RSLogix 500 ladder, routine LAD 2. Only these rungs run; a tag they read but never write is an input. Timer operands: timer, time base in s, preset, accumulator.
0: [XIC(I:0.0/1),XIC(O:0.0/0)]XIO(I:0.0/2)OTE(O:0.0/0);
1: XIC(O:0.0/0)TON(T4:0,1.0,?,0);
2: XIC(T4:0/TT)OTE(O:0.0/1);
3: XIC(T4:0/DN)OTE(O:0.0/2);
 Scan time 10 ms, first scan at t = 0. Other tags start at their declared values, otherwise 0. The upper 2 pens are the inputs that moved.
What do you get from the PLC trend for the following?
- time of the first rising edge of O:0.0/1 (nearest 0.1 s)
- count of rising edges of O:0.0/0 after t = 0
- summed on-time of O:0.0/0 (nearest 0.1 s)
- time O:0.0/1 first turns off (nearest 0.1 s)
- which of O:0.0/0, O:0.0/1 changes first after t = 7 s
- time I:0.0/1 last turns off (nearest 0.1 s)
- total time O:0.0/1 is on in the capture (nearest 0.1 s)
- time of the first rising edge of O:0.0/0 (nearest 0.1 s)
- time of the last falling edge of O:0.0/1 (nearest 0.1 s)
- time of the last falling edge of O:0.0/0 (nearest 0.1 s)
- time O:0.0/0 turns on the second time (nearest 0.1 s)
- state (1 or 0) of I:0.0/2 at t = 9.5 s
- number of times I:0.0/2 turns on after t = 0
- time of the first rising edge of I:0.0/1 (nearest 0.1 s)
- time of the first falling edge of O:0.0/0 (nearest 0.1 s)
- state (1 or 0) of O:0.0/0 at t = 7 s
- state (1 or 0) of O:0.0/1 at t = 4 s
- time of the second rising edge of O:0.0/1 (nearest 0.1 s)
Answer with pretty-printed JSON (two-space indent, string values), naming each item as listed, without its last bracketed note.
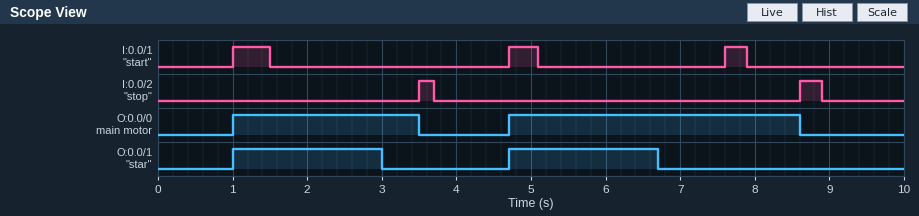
{
  "time of the first rising edge of O:0.0/1": "1.0 s",
  "count of rising edges of O:0.0/0 after t = 0": "2",
  "summed on-time of O:0.0/0": "6.4 s",
  "time O:0.0/1 first turns off": "3.0 s",
  "which of O:0.0/0, O:0.0/1 changes first after t = 7 s": "O:0.0/0",
  "time I:0.0/1 last turns off": "7.9 s",
  "total time O:0.0/1 is on in the capture": "4.0 s",
  "time of the first rising edge of O:0.0/0": "1.0 s",
  "time of the last falling edge of O:0.0/1": "6.7 s",
  "time of the last falling edge of O:0.0/0": "8.6 s",
  "time O:0.0/0 turns on the second time": "4.7 s",
  "state (1 or 0) of I:0.0/2 at t = 9.5 s": "0",
  "number of times I:0.0/2 turns on after t = 0": "2",
  "time of the first rising edge of I:0.0/1": "1.0 s",
  "time of the first falling edge of O:0.0/0": "3.5 s",
  "state (1 or 0) of O:0.0/0 at t = 7 s": "1",
  "state (1 or 0) of O:0.0/1 at t = 4 s": "0",
  "time of the second rising edge of O:0.0/1": "4.7 s"
}
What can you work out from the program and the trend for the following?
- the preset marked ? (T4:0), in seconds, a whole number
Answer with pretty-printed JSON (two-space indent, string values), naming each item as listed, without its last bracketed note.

{
  "the preset marked ? (T4:0), in seconds, a whole number": "2 s"
}
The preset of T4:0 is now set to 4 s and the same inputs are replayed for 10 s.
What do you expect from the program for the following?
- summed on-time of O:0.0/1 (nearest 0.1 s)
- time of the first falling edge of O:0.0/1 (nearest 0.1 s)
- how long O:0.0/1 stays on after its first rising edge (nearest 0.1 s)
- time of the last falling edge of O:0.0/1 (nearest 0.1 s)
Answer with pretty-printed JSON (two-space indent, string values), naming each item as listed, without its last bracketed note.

{
  "summed on-time of O:0.0/1": "6.4 s",
  "time of the first falling edge of O:0.0/1": "3.5 s",
  "how long O:0.0/1 stays on after its first rising edge": "2.5 s",
  "time of the last falling edge of O:0.0/1": "8.6 s"
}
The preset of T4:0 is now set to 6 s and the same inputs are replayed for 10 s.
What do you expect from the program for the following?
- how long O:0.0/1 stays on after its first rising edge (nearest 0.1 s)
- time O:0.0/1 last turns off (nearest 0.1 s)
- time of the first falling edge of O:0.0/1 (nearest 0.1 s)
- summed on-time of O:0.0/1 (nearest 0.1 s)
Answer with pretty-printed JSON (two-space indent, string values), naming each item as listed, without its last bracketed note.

{
  "how long O:0.0/1 stays on after its first rising edge": "2.5 s",
  "time O:0.0/1 last turns off": "8.6 s",
  "time of the first falling edge of O:0.0/1": "3.5 s",
  "summed on-time of O:0.0/1": "6.4 s"
}
